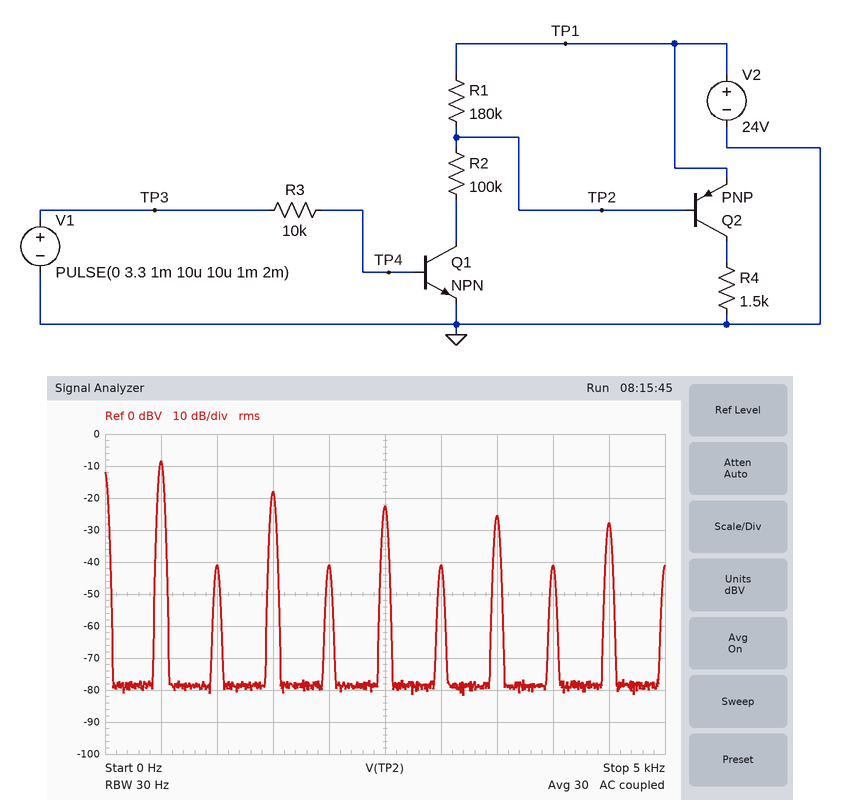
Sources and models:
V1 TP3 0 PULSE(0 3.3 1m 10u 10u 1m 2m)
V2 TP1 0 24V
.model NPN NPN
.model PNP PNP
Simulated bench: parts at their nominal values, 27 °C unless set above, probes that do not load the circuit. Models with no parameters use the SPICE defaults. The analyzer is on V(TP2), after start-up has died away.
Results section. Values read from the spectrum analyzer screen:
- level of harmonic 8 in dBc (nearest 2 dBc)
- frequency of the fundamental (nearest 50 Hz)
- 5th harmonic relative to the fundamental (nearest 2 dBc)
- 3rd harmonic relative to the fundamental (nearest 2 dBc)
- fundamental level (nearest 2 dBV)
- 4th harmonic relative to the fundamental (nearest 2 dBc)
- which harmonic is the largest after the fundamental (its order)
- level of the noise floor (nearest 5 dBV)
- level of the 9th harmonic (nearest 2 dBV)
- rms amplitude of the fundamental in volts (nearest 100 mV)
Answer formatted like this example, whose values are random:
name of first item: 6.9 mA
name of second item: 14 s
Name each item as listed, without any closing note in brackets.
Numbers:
level of harmonic 8 in dBc: -32 dBc
frequency of the fundamental: 500 Hz
5th harmonic relative to the fundamental: -14 dBc
3rd harmonic relative to the fundamental: -10 dBc
fundamental level: -8 dBV
4th harmonic relative to the fundamental: -32 dBc
which harmonic is the largest after the fundamental: 3
level of the noise floor: -80 dBV
level of the 9th harmonic: -28 dBV
rms amplitude of the fundamental in volts: 400 mV
